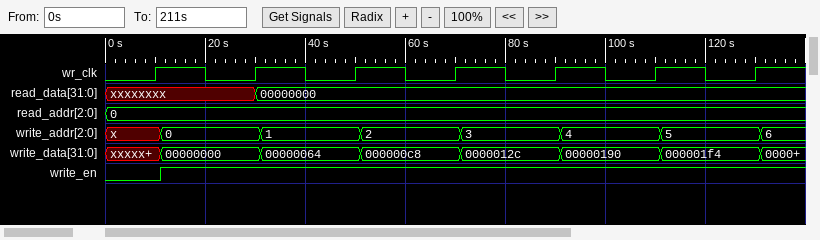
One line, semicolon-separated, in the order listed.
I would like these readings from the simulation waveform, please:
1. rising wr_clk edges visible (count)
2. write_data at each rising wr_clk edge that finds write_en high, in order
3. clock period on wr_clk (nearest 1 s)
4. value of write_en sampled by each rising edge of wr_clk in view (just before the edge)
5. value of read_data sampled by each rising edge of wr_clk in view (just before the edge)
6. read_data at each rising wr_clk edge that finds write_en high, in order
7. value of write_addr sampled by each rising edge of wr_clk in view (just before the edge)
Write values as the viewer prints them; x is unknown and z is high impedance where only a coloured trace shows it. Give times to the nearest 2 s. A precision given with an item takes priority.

7; 00000000, 00000064, 000000c8, 0000012c, 00000190, 000001f4; 20 s; 0 1 1 1 1 1 1; xxxxxxxx, xxxxxxxx, 00000000, 00000000, 00000000, 00000000, 00000000; xxxxxxxx, 00000000, 00000000, 00000000, 00000000, 00000000; x, 0, 1, 2, 3, 4, 5
